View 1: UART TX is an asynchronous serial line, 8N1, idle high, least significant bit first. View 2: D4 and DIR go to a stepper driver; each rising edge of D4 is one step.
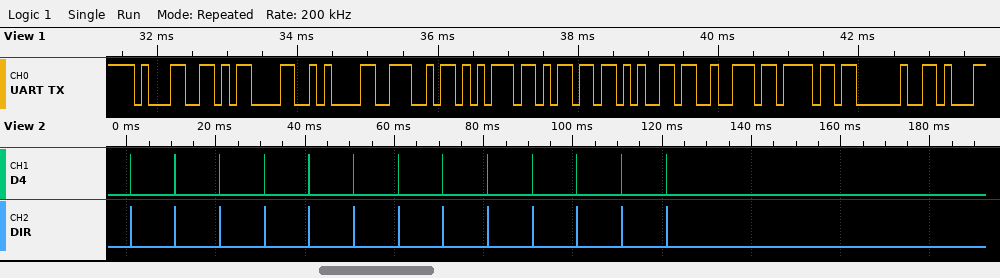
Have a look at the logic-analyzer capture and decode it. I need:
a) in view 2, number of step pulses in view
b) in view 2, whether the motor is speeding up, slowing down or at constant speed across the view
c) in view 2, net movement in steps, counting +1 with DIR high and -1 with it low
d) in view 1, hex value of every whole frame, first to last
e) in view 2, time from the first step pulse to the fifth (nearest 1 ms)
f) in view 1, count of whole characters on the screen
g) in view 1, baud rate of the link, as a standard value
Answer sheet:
13
constant speed
+13
31 0D 0A 4E 75 6D 65 72 6F 20
40 ms
10
9600 baud
